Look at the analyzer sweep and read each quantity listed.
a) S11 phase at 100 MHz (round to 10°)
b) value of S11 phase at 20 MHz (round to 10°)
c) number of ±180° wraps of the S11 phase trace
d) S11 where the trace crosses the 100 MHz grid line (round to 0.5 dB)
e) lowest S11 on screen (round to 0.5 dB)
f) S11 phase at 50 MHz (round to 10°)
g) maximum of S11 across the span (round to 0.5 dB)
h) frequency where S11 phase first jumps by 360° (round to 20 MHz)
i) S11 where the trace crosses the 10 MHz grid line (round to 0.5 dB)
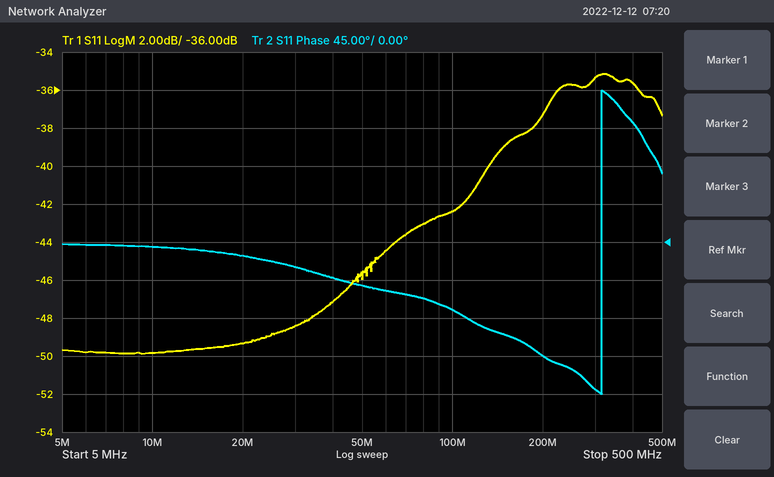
-80°
-20°
1
-42.5 dB
-50.0 dB
-50°
-35.0 dB
320 MHz
-50.0 dB
